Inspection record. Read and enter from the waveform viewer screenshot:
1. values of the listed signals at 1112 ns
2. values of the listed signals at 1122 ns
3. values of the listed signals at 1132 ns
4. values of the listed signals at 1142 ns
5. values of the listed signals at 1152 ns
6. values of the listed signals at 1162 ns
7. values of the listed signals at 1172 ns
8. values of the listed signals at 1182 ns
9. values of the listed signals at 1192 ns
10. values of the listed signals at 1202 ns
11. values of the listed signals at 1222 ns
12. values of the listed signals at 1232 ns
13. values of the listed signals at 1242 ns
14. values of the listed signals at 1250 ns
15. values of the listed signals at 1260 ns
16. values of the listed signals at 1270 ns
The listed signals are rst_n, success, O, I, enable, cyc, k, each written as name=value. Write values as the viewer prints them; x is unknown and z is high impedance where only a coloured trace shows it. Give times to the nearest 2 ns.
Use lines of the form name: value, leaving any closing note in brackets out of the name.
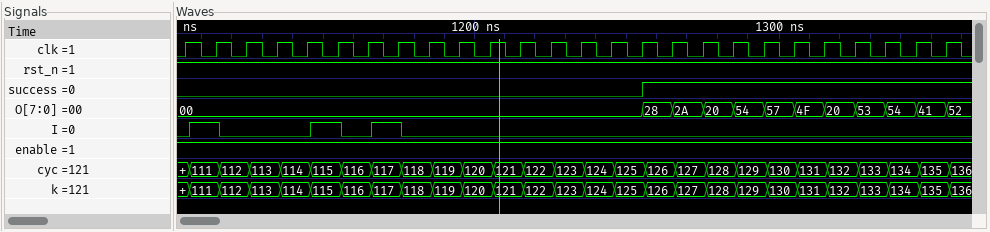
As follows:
values of the listed signals at 1112 ns: rst_n=1, success=0, O=00, I=1, enable=1, cyc=111, k=111
values of the listed signals at 1122 ns: rst_n=1, success=0, O=00, I=0, enable=1, cyc=112, k=112
values of the listed signals at 1132 ns: rst_n=1, success=0, O=00, I=0, enable=1, cyc=113, k=113
values of the listed signals at 1142 ns: rst_n=1, success=0, O=00, I=0, enable=1, cyc=114, k=114
values of the listed signals at 1152 ns: rst_n=1, success=0, O=00, I=1, enable=1, cyc=115, k=115
values of the listed signals at 1162 ns: rst_n=1, success=0, O=00, I=0, enable=1, cyc=116, k=116
values of the listed signals at 1172 ns: rst_n=1, success=0, O=00, I=1, enable=1, cyc=117, k=117
values of the listed signals at 1182 ns: rst_n=1, success=0, O=00, I=0, enable=1, cyc=118, k=118
values of the listed signals at 1192 ns: rst_n=1, success=0, O=00, I=0, enable=1, cyc=119, k=119
values of the listed signals at 1202 ns: rst_n=1, success=0, O=00, I=0, enable=1, cyc=120, k=120
values of the listed signals at 1222 ns: rst_n=1, success=0, O=00, I=0, enable=1, cyc=122, k=122
values of the listed signals at 1232 ns: rst_n=1, success=0, O=00, I=0, enable=1, cyc=123, k=123
values of the listed signals at 1242 ns: rst_n=1, success=0, O=00, I=0, enable=1, cyc=124, k=124
values of the listed signals at 1250 ns: rst_n=1, success=0, O=00, I=0, enable=1, cyc=125, k=125
values of the listed signals at 1260 ns: rst_n=1, success=1, O=28, I=0, enable=1, cyc=126, k=126
values of the listed signals at 1270 ns: rst_n=1, success=1, O=2A, I=0, enable=1, cyc=127, k=127
